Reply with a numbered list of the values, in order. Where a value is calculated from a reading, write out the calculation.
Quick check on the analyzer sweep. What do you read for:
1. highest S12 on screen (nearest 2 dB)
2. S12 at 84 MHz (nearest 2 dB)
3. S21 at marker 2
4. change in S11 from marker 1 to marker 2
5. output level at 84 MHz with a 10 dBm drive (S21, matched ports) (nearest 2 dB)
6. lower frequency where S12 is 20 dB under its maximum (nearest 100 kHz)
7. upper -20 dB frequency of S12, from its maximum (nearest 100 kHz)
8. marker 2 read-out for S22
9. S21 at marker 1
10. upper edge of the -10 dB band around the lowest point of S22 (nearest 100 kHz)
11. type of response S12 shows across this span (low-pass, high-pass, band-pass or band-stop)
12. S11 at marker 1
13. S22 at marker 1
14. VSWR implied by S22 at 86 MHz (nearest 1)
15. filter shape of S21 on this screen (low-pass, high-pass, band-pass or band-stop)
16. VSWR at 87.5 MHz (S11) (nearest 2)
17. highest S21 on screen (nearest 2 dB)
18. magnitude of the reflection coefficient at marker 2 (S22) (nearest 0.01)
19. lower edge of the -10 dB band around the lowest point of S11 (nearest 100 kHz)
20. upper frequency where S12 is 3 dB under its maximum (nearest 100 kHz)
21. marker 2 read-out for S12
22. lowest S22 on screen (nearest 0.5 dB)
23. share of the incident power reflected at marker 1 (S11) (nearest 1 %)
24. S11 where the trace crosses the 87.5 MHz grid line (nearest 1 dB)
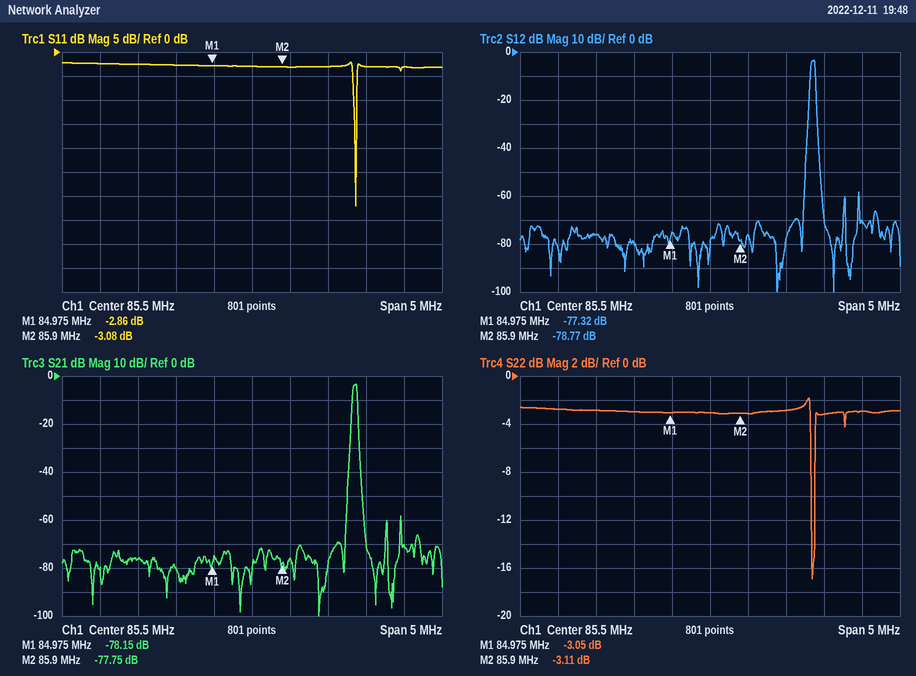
1. -4 dB
2. -76 dB
3. -77.75 dB
4. -3.08 − (-2.86) = -0.22 dB
5. 10 dBm + (-76 dB) = -66 dBm
6. 86.8 MHz
7. 86.9 MHz
8. -3.11 dB
9. -78.15 dB
10. 86.9 MHz
11. band-pass
12. -2.86 dB
13. -3.05 dB
14. |Γ| = 10^(-3/20) = 0.7079; VSWR = (1 + 0.7079)/(1 − 0.7079) ≈ 6
15. band-pass
16. |Γ| = 10^(-3/20) = 0.7079; VSWR = (1 + 0.7079)/(1 − 0.7079) ≈ 6
17. -4 dB
18. 10^(-3.11/20) ≈ 0.70
19. 86.8 MHz
20. 86.9 MHz
21. -78.77 dB
22. -17.0 dB
23. 10^(-2.86/10) ≈ 52 %
24. -3 dB
